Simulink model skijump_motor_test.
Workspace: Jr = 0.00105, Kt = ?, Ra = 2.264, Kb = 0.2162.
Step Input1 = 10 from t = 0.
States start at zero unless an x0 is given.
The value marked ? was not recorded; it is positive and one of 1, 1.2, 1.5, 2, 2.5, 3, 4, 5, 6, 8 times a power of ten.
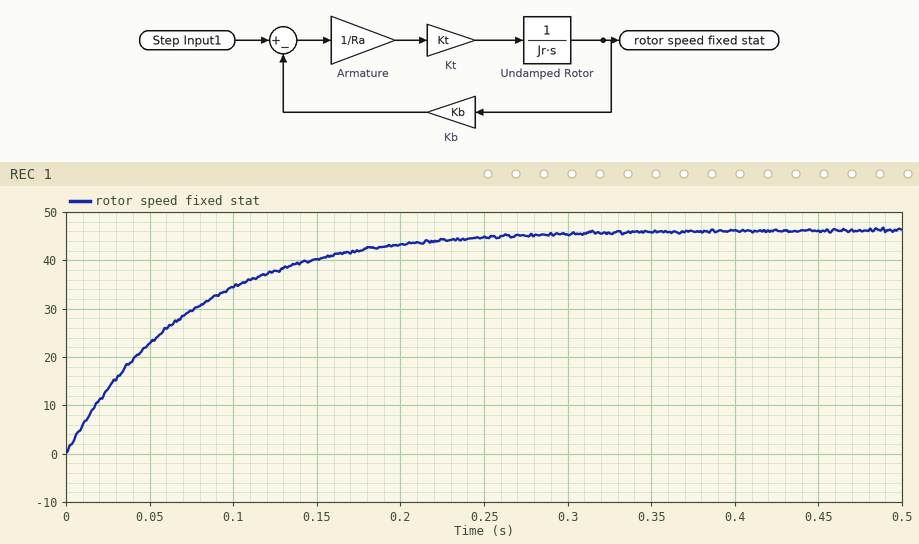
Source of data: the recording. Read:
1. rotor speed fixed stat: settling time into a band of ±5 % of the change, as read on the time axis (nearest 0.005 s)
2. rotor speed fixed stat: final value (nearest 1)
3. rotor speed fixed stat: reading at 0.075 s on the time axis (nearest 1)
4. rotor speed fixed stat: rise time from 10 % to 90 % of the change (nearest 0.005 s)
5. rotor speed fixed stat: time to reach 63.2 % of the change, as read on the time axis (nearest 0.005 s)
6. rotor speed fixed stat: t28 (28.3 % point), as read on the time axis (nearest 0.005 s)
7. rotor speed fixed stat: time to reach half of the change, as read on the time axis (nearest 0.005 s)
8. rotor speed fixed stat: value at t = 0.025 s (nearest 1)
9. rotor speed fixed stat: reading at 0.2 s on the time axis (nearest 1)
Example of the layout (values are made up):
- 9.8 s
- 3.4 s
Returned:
- 0.220 s
- 46
- 30
- 0.160 s
- 0.075 s
- 0.025 s
- 0.050 s
- 13
- 43
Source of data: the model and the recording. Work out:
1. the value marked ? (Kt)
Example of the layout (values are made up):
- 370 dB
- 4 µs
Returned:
- 0.15
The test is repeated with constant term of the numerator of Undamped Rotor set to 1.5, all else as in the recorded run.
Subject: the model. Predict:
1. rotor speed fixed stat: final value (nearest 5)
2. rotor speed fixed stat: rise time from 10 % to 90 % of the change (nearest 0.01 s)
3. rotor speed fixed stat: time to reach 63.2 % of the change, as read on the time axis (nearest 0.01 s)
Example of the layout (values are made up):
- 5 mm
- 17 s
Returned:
- 45
- 0.11 s
- 0.05 s
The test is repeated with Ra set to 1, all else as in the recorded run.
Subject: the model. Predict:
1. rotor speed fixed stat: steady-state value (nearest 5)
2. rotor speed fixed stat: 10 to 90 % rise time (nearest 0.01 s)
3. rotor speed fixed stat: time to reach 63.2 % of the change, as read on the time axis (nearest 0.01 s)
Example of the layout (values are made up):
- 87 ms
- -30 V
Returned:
- 45
- 0.07 s
- 0.03 s
